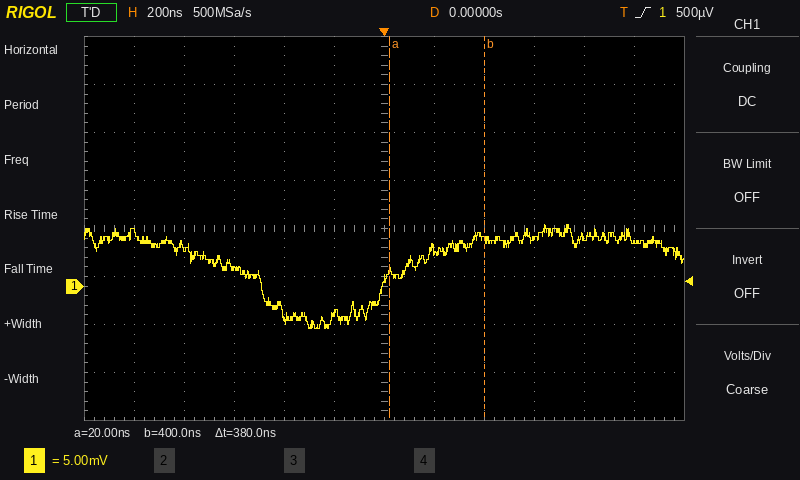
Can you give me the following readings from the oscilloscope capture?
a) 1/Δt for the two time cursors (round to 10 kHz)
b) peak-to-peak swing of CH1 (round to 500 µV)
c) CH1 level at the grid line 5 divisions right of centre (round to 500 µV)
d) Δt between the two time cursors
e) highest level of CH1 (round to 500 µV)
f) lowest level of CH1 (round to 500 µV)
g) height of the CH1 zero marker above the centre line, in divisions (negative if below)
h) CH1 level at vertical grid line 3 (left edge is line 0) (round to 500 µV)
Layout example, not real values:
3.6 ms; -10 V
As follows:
2.63 MHz; 11.0 mV; 4.5 mV; 380 ns; 6.5 mV; -4.5 mV; -1.2 div; 2.0 mV
